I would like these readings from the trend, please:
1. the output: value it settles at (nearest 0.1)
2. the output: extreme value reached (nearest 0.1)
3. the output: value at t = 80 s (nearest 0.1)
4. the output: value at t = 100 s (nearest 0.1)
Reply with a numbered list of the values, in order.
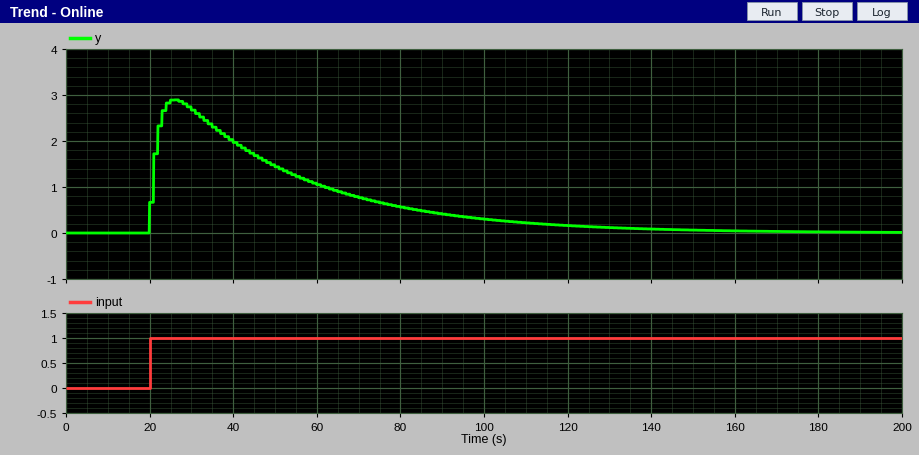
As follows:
1. 0.0
2. 2.9
3. 0.6
4. 0.3
